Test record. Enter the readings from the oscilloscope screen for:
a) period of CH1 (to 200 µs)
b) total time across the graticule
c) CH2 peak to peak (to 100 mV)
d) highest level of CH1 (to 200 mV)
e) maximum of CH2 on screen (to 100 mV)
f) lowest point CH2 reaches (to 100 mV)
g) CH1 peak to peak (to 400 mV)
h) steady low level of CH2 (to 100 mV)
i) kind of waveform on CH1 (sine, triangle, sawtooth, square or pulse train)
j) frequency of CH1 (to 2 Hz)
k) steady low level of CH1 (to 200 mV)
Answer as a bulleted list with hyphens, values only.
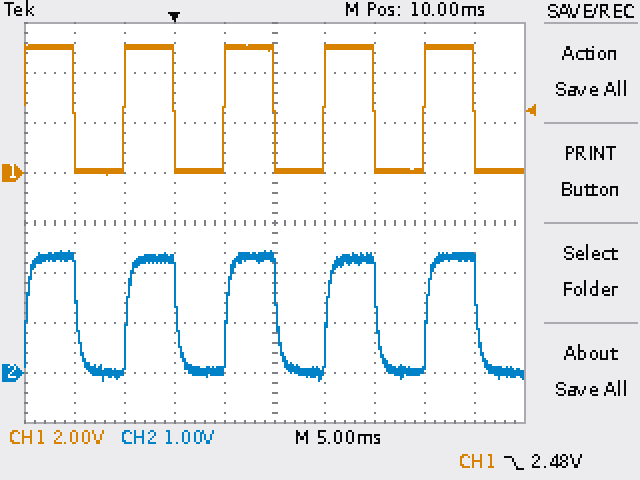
- 10.0 ms
- 50 ms
- 2.6 V
- 5.2 V
- 2.4 V
- -200 mV
- 5.2 V
- 0.0 V
- square
- 100 Hz
- 0.0 V
